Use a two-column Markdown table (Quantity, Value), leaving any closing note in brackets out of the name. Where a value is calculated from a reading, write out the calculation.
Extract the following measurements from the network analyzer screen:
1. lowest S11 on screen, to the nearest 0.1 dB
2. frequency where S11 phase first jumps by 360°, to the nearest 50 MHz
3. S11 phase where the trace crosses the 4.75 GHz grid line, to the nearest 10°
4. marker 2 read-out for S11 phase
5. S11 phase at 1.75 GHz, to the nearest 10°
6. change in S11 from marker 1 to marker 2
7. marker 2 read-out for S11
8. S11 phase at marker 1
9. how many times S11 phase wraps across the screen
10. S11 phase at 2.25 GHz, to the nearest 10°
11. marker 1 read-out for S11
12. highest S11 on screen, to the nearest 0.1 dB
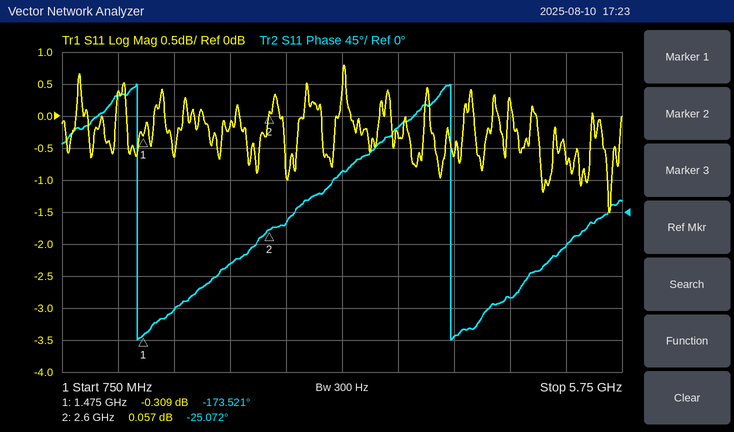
| Quantity | Value |
|---|---|
| lowest S11 on screen, to the nearest 0.1 dB | -1.5 dB |
| frequency where S11 phase first jumps by 360°, to the nearest 50 MHz | 1.40 GHz |
| S11 phase where the trace crosses the 4.75 GHz grid line, to the nearest 10° | -120° |
| marker 2 read-out for S11 phase | -25.072° |
| S11 phase at 1.75 GHz, to the nearest 10° | -140° |
| change in S11 from marker 1 to marker 2 | 0.057 − (-0.309) = 0.366 dB |
| marker 2 read-out for S11 | 0.057 dB |
| S11 phase at marker 1 | -173.521° |
| how many times S11 phase wraps across the screen | 2 |
| S11 phase at 2.25 GHz, to the nearest 10° | -70° |
| marker 1 read-out for S11 | -0.309 dB |
| highest S11 on screen, to the nearest 0.1 dB | 0.8 dB |
